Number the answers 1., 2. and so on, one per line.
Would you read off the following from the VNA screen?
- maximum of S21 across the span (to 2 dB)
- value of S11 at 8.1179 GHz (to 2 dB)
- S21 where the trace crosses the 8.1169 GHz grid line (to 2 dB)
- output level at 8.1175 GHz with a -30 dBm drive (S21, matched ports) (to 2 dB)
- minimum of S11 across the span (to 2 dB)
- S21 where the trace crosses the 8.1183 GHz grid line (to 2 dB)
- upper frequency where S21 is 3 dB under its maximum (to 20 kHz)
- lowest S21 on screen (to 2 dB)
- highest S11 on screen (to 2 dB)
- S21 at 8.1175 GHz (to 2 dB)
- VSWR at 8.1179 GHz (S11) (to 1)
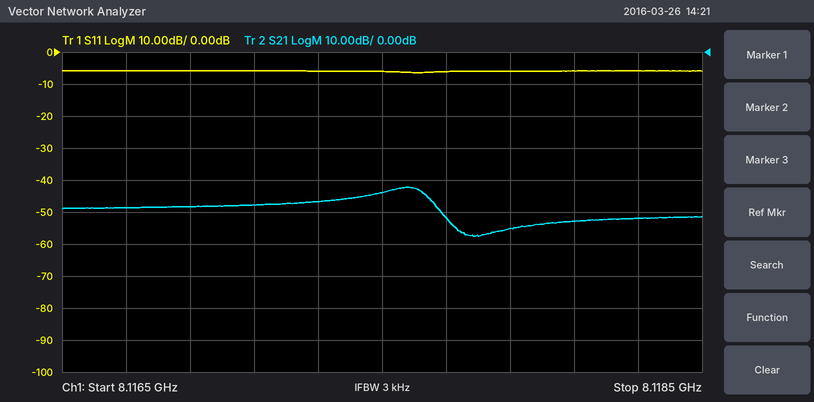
1. -42 dB
2. -6 dB
3. -48 dB
4. -74 dBm
5. -6 dB
6. -52 dB
7. 8.11764 GHz
8. -58 dB
9. -6 dB
10. -44 dB
11. 3
